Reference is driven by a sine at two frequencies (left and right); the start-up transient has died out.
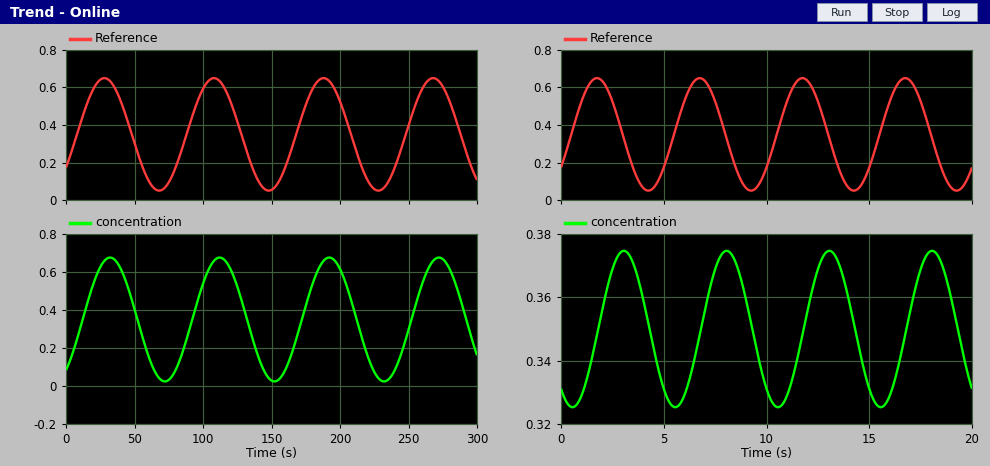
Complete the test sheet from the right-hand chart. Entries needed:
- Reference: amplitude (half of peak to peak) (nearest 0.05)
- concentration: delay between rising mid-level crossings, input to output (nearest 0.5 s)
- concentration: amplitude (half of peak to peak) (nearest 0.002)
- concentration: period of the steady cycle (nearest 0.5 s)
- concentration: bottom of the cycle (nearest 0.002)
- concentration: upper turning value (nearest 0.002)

0.30
1.5 s
0.024
5.0 s
0.326
0.374
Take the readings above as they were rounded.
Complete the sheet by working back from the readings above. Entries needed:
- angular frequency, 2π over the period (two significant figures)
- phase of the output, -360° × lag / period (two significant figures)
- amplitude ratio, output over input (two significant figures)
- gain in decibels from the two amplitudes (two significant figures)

1.3 rad/s
-110°
0.080
-22 dB
